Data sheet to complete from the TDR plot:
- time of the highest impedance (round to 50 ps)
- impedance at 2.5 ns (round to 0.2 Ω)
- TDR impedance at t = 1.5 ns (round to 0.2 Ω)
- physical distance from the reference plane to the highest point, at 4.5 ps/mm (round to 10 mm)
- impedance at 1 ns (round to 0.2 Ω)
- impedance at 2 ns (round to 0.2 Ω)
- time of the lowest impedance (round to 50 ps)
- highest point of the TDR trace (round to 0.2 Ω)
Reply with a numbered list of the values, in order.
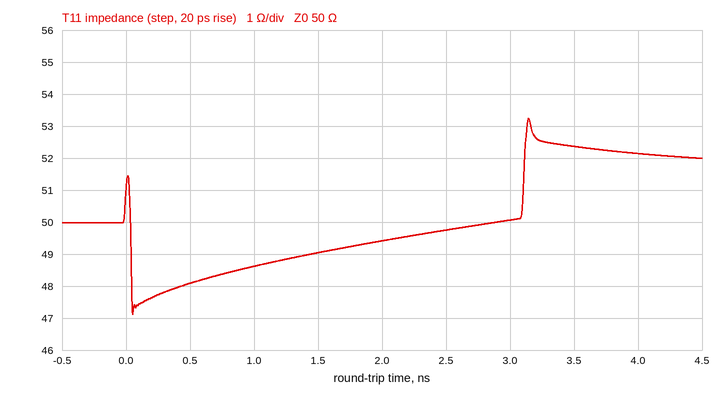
1. 3.15 ns
2. 49.8 Ω
3. 49.0 Ω
4. 350 mm
5. 48.6 Ω
6. 49.4 Ω
7. 50 ps
8. 53.2 Ω
